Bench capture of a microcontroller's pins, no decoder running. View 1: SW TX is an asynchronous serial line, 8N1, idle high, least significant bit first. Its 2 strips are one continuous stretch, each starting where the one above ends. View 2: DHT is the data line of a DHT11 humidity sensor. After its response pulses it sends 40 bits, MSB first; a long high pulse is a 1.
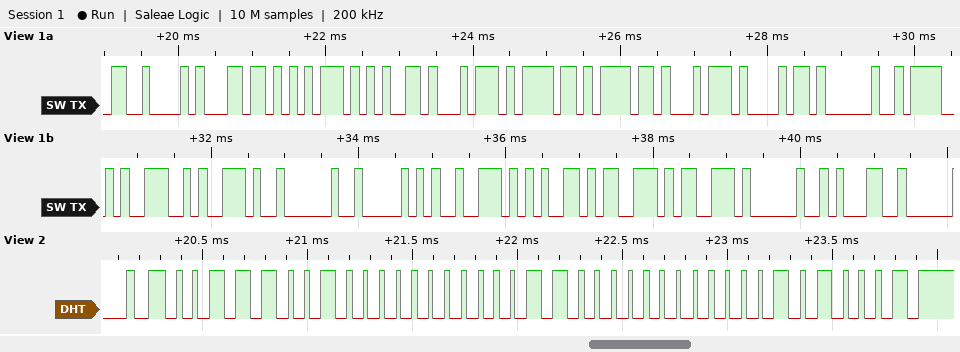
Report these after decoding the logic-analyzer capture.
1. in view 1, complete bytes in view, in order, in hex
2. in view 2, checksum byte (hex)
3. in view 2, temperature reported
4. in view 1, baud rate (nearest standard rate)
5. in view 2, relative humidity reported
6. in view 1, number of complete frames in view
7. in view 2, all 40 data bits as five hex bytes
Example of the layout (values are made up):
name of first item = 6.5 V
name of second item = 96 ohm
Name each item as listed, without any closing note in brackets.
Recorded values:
in view 1, complete bytes in view, in order, in hex = 42 6C 75 65 74 6F 6F 74 68 20 4F 4E 2E 20 50 72 65 73 73 20 31
in view 2, checksum byte = 0x51
in view 2, temperature reported = 24.0 °C
in view 1, baud rate = 9600 baud
in view 2, relative humidity reported = 57 %
in view 1, number of complete frames in view = 21
in view 2, all 40 data bits as five hex bytes = 39 00 18 00 51
